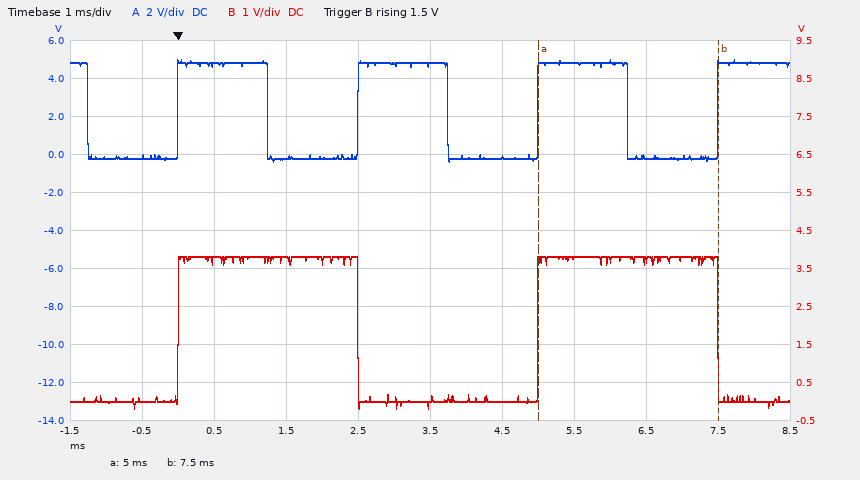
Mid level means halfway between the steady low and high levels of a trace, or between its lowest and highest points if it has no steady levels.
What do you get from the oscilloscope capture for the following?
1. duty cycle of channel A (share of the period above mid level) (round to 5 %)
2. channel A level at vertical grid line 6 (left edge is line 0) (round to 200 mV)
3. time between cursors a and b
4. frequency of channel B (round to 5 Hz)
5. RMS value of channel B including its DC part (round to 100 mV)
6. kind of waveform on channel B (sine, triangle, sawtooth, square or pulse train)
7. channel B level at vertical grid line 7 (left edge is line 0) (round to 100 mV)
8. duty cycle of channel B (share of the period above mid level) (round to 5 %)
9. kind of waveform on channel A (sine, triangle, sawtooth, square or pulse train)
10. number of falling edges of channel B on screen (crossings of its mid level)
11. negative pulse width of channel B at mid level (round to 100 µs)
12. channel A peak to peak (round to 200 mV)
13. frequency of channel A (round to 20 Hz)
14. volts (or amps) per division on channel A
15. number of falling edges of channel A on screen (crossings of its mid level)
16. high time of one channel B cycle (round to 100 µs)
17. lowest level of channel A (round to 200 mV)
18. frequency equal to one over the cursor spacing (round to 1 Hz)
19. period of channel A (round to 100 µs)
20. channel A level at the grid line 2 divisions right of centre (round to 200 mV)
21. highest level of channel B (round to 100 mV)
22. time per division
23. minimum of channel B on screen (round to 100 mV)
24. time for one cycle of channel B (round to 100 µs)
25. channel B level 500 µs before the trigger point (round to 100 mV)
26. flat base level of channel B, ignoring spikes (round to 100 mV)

50 %
-200 mV
2.5 ms
200 Hz
2.7 V
square
3.8 V
50 %
square
2
2.5 ms
5.4 V
400 Hz
2 V
4
2.5 ms
-400 mV
400 Hz
2.5 ms
4.8 V
3.8 V
1 ms
-200 mV
5.0 ms
0.0 V
0.0 V
